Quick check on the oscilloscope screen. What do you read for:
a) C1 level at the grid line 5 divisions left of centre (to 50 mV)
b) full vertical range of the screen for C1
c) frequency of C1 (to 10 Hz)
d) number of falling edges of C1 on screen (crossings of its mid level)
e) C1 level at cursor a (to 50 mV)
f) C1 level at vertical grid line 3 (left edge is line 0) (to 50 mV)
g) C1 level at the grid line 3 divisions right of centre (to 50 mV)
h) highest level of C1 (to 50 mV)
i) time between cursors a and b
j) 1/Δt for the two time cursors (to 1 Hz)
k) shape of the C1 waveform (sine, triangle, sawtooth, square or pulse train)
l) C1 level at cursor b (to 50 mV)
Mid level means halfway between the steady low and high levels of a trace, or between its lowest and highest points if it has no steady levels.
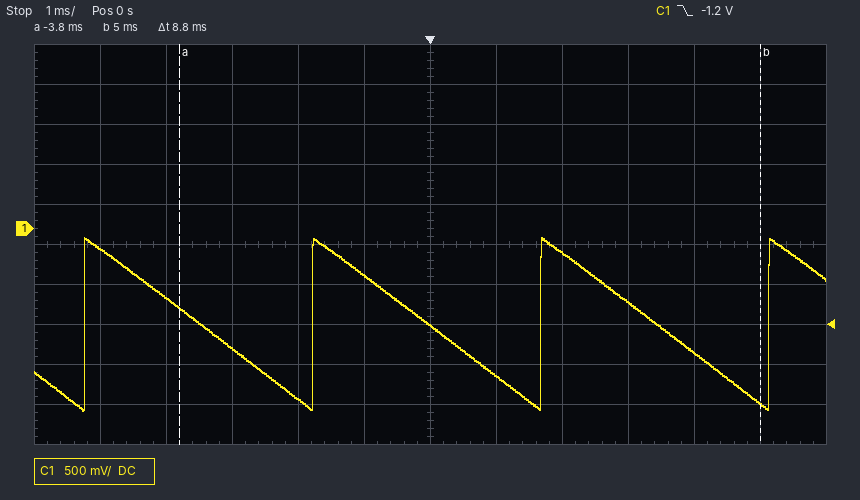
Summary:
-250 mV
5 V
290 Hz
3
-1.00 V
-1.50 V
-900 mV
-100 mV
8.8 ms
114 Hz
sawtooth
-2.20 V
